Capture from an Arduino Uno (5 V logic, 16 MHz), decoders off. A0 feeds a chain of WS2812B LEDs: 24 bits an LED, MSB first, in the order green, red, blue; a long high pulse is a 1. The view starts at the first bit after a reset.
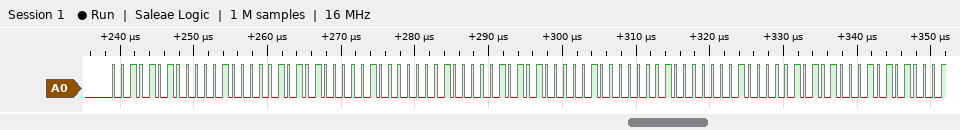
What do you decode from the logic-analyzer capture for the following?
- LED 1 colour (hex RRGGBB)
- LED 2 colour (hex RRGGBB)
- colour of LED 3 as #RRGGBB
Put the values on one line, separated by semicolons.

#082A2A; #08082A; #080808
